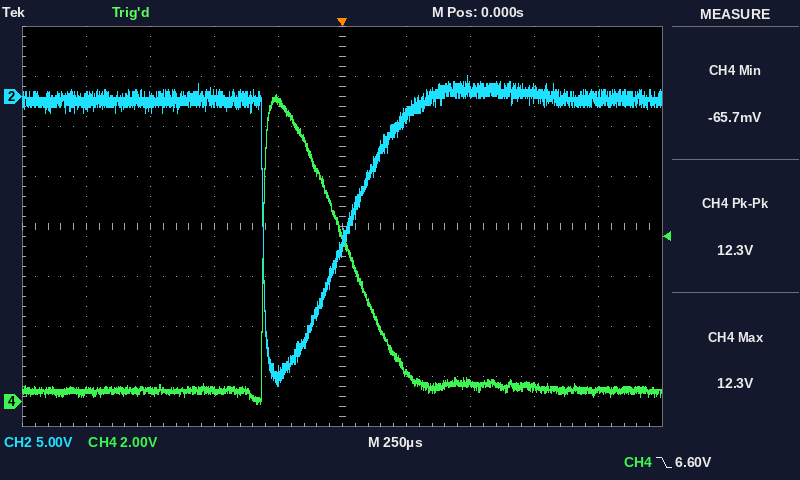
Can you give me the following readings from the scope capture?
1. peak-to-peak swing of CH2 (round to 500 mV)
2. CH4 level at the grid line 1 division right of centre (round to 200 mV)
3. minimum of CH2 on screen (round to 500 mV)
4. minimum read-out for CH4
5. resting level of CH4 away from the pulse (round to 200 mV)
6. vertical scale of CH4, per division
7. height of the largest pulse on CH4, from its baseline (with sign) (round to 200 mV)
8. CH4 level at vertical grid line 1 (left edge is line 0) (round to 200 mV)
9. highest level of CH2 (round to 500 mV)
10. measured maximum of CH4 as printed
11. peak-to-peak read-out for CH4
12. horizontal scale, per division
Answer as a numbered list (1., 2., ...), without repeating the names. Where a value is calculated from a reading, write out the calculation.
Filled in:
1. 2.0 V − (-29.0 V) = 31.0 V
2. 1.2 V
3. -29.0 V
4. -65.7 mV
5. 400 mV
6. 2 V
7. +11.8 V
8. 400 mV
9. 2.0 V
10. 12.3 V
11. 12.3 V
12. 250 µs
